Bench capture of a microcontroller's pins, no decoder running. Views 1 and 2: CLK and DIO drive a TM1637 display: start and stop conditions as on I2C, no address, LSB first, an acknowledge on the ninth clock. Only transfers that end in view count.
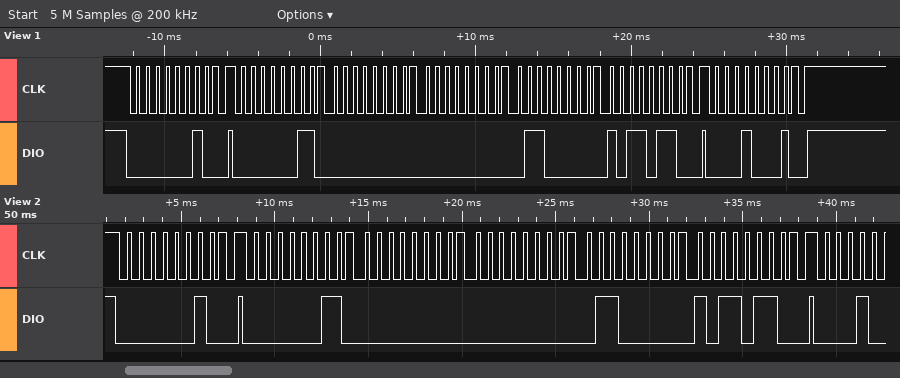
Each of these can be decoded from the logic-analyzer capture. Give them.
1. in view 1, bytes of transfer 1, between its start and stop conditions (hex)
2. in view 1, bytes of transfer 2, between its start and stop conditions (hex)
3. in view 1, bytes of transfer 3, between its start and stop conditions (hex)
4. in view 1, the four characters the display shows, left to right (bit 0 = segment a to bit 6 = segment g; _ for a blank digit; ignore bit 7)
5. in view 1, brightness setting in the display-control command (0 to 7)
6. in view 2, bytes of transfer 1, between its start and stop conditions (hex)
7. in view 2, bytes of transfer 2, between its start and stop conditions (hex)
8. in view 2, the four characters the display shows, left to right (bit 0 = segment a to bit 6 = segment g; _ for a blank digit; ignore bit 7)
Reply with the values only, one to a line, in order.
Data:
40
C0 00 00 06 6D
88
__15
0
40
C0 00 00 06 6D
__15
